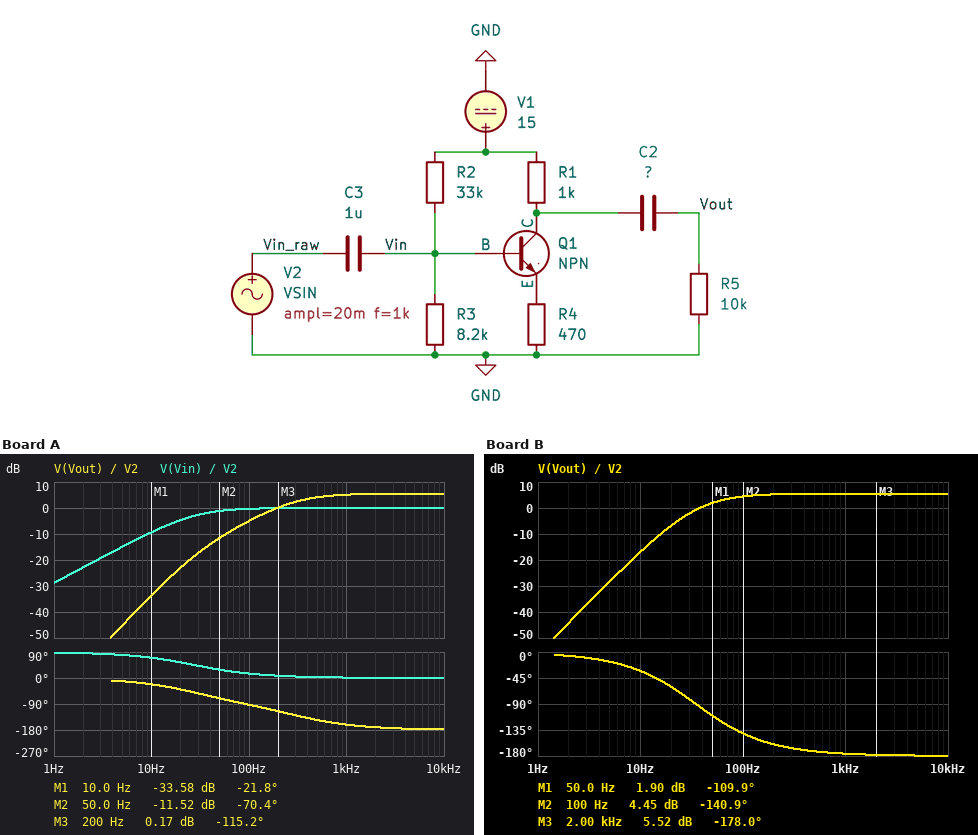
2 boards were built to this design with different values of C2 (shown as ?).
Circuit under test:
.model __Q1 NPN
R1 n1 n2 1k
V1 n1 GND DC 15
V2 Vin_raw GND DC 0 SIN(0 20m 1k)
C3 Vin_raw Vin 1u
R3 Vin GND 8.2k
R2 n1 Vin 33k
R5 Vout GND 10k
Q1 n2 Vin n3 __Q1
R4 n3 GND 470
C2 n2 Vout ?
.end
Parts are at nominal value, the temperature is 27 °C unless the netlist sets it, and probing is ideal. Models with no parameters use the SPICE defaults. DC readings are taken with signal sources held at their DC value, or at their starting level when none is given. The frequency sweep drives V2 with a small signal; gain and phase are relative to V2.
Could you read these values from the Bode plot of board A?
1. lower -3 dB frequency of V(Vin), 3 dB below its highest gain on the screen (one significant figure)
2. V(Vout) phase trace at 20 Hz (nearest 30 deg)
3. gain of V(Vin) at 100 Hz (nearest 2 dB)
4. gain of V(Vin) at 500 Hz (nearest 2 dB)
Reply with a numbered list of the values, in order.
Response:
1. 30 Hz
2. -30 deg
3. 0 dB
4. 0 dB
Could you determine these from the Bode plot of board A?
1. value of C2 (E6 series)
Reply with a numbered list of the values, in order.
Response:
1. 47 nF
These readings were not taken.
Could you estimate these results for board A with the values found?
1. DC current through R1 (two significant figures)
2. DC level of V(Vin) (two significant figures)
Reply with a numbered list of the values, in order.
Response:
1. 4.0 mA
2. 2.7 V
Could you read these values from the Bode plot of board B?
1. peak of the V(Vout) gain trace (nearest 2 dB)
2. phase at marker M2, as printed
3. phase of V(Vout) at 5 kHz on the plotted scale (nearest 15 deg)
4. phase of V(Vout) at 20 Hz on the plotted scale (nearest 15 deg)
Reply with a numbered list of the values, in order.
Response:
1. 6 dB
2. -140.9 deg
3. -180 deg
4. -60 deg
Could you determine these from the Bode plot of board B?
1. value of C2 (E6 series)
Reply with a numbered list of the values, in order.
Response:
1. 330 nF
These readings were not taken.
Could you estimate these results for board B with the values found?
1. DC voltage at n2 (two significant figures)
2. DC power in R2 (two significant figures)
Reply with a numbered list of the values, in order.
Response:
1. 11 V
2. 4.6 mW
